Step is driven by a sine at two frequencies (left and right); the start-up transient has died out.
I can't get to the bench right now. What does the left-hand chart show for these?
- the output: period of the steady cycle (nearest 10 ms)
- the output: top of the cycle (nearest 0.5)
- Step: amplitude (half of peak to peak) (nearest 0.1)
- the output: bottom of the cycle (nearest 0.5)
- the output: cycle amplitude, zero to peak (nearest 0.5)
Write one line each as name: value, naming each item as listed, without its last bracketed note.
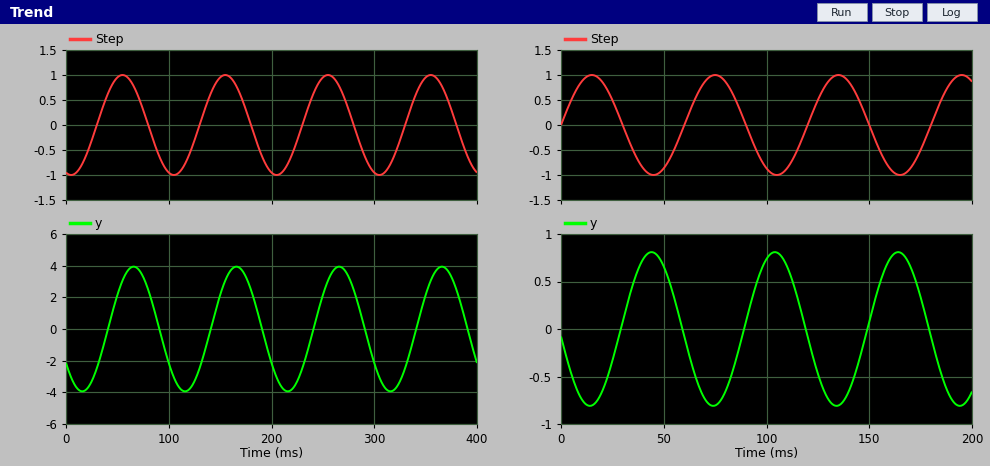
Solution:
the output: period of the steady cycle: 100 ms
the output: top of the cycle: 4.0
Step: amplitude (half of peak to peak): 1.0
the output: bottom of the cycle: -4.0
the output: cycle amplitude, zero to peak: 4.0
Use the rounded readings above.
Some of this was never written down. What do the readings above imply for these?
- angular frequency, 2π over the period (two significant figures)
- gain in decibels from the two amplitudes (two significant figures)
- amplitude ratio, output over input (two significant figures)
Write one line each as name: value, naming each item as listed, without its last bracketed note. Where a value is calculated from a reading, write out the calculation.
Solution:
angular frequency, 2π over the period: 2π / 100 = 0.063 rad/ms
gain in decibels from the two amplitudes: 20 log10(4 / 1) = 12 dB
amplitude ratio, output over input: 4 / 1 = 4.0
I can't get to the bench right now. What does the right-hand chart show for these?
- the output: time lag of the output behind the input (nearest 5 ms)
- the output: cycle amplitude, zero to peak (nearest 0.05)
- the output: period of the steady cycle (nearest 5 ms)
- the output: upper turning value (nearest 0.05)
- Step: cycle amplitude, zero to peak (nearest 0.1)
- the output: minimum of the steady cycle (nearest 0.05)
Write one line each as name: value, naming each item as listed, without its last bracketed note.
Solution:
the output: time lag of the output behind the input: 30 ms
the output: cycle amplitude, zero to peak: 0.80
the output: period of the steady cycle: 60 ms
the output: upper turning value: 0.80
Step: cycle amplitude, zero to peak: 1.0
the output: minimum of the steady cycle: -0.80
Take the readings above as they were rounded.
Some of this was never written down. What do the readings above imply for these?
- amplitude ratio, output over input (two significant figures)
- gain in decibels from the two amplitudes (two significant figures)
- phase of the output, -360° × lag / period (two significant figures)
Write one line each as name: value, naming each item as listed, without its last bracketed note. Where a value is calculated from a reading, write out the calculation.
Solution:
amplitude ratio, output over input: 0.8 / 1 = 0.80
gain in decibels from the two amplitudes: 20 log10(0.8 / 1) = -1.9 dB
phase of the output, -360° × lag / period: -360 × 30 / 60 = -180°
